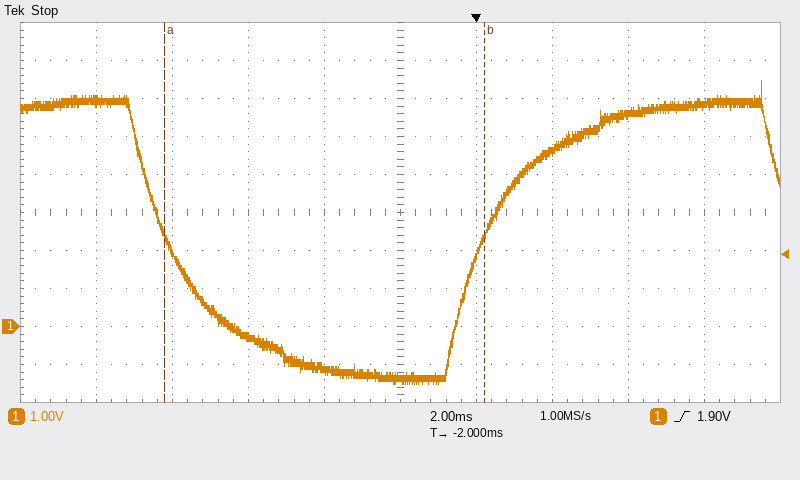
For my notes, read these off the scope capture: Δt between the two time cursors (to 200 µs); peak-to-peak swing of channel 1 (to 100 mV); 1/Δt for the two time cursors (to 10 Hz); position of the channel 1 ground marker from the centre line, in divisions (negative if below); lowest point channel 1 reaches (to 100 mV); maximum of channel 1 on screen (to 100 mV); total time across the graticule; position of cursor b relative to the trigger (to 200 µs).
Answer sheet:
8.4 ms
8.0 V
120 Hz
-3.0 div
-1.5 V
6.5 V
20 ms
+200 µs
